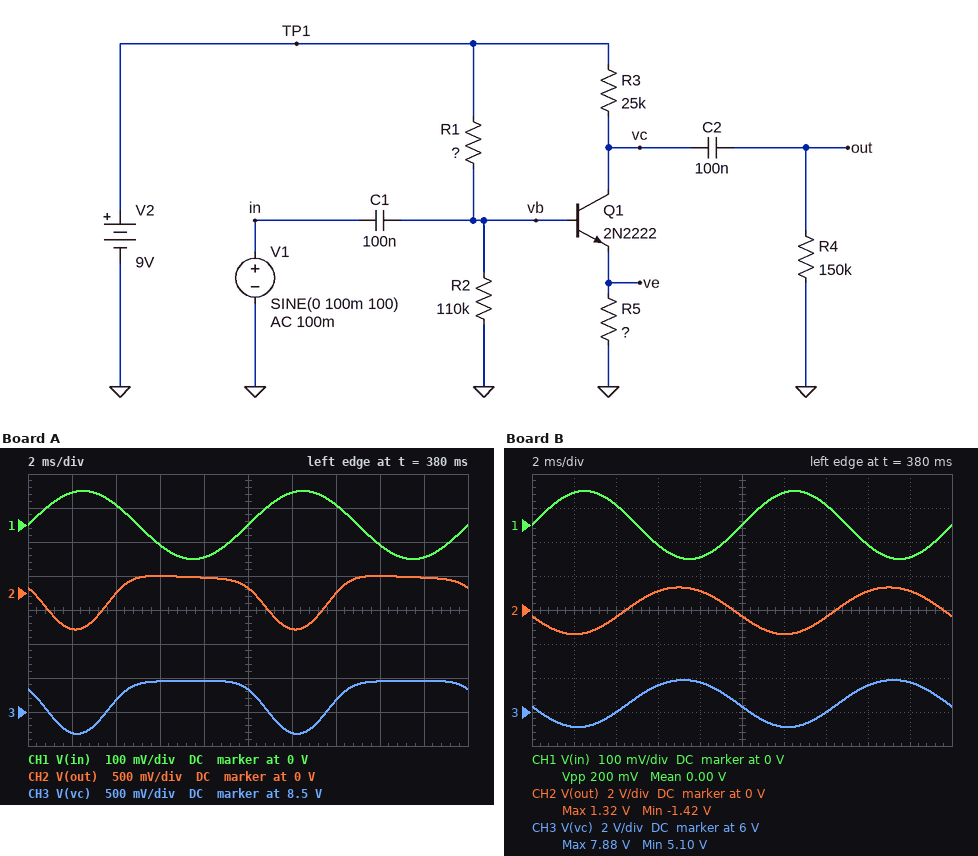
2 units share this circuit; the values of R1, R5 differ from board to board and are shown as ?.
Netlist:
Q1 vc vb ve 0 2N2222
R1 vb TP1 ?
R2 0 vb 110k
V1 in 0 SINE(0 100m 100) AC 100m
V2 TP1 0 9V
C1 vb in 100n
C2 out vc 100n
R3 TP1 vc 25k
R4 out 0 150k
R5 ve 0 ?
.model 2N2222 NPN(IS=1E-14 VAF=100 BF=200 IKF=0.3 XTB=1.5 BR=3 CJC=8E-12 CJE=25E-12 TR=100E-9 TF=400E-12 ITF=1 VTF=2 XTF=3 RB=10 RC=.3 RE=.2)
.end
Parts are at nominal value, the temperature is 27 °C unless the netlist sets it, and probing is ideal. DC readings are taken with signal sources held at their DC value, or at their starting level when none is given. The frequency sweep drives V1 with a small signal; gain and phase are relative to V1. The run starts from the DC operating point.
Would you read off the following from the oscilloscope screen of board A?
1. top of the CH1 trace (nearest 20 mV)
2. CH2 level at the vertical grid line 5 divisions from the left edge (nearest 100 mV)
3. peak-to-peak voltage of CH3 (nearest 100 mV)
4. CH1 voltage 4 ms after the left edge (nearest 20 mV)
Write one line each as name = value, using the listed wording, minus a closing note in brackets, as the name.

top of the CH1 trace = 100 mV
CH2 level at the vertical grid line 5 divisions from the left edge = 100 mV
peak-to-peak voltage of CH3 = 800 mV
CH1 voltage 4 ms after the left edge = 60 mV
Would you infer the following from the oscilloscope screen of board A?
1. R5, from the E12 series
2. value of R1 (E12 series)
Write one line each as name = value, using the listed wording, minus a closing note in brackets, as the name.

R5, from the E12 series = 1.2 kΩ
value of R1 = 1.8 MΩ
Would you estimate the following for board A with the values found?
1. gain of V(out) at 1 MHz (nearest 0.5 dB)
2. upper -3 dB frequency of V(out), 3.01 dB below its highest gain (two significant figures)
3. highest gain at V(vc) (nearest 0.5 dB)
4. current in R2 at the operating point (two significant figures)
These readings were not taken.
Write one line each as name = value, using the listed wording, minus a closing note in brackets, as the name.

gain of V(out) at 1 MHz = 8.5 dB
upper -3 dB frequency of V(out), 3.01 dB below its highest gain = 2.7 MHz
highest gain at V(vc) = 9.0 dB
current in R2 at the operating point = 4.7 µA
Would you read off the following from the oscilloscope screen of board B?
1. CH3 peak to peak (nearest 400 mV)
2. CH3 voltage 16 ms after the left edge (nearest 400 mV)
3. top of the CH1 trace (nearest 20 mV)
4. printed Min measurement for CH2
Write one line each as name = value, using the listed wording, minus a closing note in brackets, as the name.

CH3 peak to peak = 2.8 V
CH3 voltage 16 ms after the left edge = 7.6 V
top of the CH1 trace = 100 mV
printed Min measurement for CH2 = -1.42 V
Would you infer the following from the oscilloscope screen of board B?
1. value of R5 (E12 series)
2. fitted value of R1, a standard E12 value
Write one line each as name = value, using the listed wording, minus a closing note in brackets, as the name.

value of R5 = 1.2 kΩ
fitted value of R1, a standard E12 value = 1.2 MΩ
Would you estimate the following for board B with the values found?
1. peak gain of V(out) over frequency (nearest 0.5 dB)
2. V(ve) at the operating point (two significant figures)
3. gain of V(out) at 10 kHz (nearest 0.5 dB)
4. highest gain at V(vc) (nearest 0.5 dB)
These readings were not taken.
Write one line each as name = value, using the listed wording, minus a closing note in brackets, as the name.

peak gain of V(out) over frequency = 23.0 dB
V(ve) at the operating point = 120 mV
gain of V(out) at 10 kHz = 23.0 dB
highest gain at V(vc) = 23.0 dB
